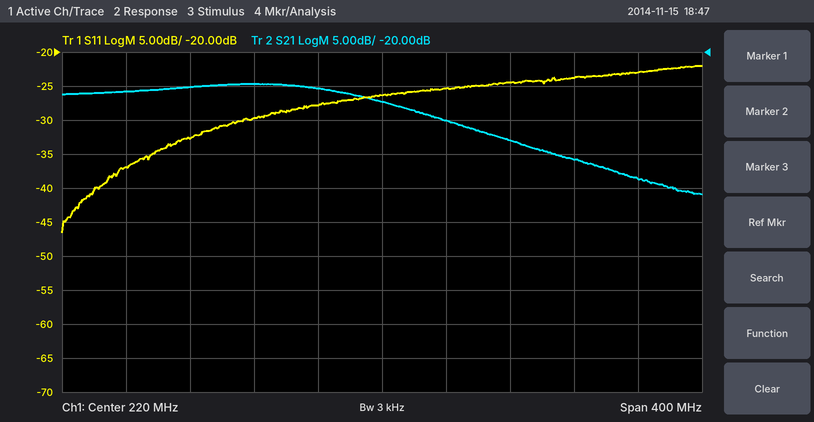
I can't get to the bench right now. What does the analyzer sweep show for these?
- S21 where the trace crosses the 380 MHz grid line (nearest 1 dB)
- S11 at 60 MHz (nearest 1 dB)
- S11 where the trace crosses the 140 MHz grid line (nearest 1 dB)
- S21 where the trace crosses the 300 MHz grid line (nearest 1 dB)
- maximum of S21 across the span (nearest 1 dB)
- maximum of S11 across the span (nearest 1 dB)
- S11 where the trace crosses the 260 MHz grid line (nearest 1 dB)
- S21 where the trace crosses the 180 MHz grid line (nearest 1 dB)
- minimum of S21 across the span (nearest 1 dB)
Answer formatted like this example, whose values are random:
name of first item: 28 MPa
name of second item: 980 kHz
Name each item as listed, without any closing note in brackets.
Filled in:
S21 where the trace crosses the 380 MHz grid line: -39 dB
S11 at 60 MHz: -37 dB
S11 where the trace crosses the 140 MHz grid line: -30 dB
S21 where the trace crosses the 300 MHz grid line: -33 dB
maximum of S21 across the span: -25 dB
maximum of S11 across the span: -22 dB
S11 where the trace crosses the 260 MHz grid line: -25 dB
S21 where the trace crosses the 180 MHz grid line: -25 dB
minimum of S21 across the span: -41 dB
